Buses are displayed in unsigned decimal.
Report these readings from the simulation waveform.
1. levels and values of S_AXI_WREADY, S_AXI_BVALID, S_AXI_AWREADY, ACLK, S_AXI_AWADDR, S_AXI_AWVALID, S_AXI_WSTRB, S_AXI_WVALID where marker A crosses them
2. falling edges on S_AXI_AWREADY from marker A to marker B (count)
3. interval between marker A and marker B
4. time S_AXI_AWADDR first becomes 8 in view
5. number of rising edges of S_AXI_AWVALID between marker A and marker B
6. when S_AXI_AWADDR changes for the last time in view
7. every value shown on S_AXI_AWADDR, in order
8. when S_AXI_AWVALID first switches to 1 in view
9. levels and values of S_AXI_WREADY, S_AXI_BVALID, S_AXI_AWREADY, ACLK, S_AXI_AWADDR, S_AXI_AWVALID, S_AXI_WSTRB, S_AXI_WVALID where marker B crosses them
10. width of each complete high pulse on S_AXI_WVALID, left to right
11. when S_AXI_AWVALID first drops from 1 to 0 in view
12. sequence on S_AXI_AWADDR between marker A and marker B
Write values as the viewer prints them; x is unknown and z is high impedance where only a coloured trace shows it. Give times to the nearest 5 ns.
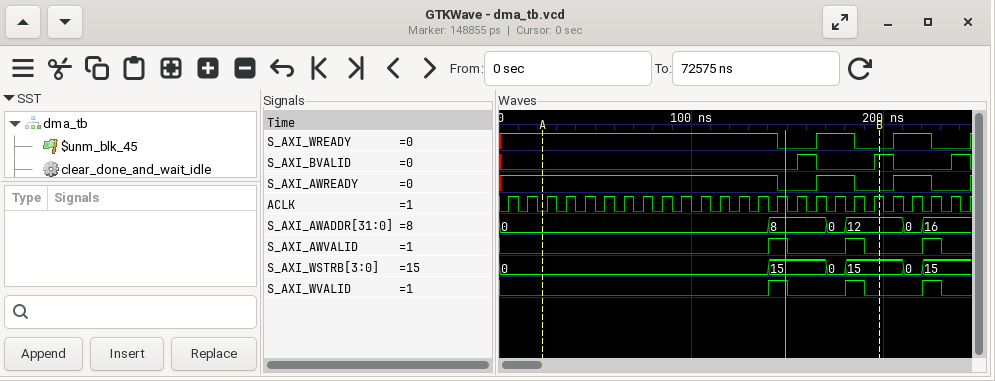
S_AXI_WREADY=1, S_AXI_BVALID=0, S_AXI_AWREADY=1, ACLK=0, S_AXI_AWADDR=0, S_AXI_AWVALID=0, S_AXI_WSTRB=0, S_AXI_WVALID=0
2
175 ns
140 ns
2
220 ns
0, 8, 0, 12, 0, 16
140 ns
S_AXI_WREADY=0, S_AXI_BVALID=1, S_AXI_AWREADY=0, ACLK=1, S_AXI_AWADDR=12, S_AXI_AWVALID=0, S_AXI_WSTRB=15, S_AXI_WVALID=0
10 ns, 10 ns, 10 ns
150 ns
0, 8, 0, 12
